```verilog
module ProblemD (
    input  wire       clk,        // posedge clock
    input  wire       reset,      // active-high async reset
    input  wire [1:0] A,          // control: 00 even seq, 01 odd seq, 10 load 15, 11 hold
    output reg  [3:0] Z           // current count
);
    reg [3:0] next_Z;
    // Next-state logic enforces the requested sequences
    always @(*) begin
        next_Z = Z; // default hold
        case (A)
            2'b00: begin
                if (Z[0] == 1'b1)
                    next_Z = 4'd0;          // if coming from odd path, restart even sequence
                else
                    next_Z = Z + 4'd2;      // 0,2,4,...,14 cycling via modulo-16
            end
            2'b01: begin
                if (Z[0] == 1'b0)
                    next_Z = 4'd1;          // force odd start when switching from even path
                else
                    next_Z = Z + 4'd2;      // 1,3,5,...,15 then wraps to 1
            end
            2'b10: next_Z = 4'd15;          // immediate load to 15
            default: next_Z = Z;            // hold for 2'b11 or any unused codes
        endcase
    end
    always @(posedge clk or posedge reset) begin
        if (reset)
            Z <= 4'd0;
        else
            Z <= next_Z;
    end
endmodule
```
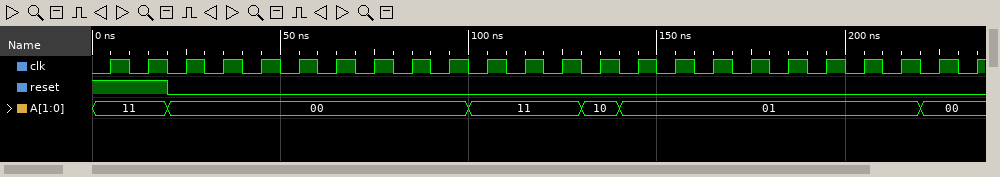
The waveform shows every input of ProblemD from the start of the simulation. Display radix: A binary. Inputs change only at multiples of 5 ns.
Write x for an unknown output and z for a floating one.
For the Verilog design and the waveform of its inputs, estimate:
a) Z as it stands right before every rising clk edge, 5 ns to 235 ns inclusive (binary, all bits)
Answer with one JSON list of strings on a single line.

["0000, 0000, 0000, 0010, 0100, 0110, 1000, 1010, 1100, 1110, 0000, 0000, 0000, 0000, 1111, 0001, 0011, 0101, 0111, 1001, 1011, 1101, 1111, 0000"]
